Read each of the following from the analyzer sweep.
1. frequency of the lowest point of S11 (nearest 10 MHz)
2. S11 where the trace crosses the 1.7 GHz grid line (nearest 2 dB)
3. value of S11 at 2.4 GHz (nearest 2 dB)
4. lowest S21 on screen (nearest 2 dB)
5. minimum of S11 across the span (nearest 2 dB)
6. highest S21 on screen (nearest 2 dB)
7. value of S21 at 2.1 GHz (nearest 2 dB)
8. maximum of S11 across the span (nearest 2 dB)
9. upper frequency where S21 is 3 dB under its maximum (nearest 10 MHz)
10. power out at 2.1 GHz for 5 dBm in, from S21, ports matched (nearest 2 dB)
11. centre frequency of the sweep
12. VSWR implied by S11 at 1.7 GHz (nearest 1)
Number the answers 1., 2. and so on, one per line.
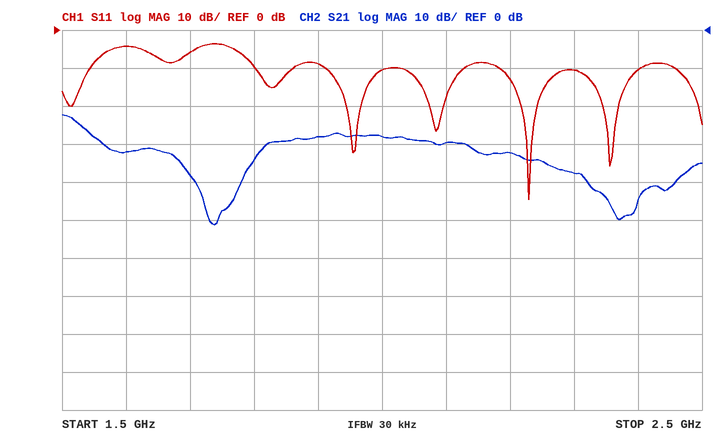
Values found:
1. 2.23 GHz
2. -6 dB
3. -10 dB
4. -52 dB
5. -44 dB
6. -22 dB
7. -30 dB
8. -4 dB
9. 1.53 GHz
10. -24 dBm
11. 2 GHz
12. 3
